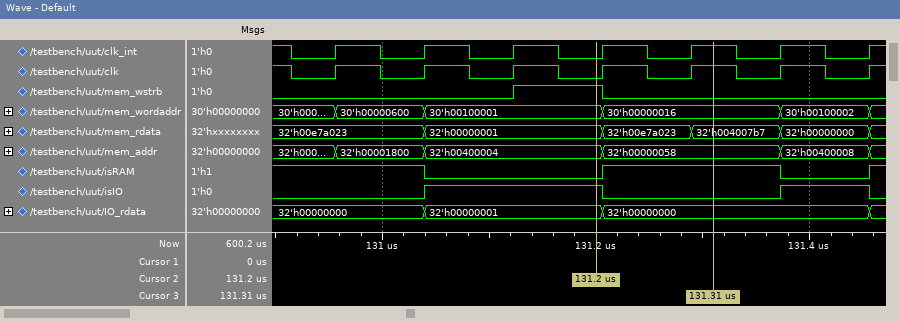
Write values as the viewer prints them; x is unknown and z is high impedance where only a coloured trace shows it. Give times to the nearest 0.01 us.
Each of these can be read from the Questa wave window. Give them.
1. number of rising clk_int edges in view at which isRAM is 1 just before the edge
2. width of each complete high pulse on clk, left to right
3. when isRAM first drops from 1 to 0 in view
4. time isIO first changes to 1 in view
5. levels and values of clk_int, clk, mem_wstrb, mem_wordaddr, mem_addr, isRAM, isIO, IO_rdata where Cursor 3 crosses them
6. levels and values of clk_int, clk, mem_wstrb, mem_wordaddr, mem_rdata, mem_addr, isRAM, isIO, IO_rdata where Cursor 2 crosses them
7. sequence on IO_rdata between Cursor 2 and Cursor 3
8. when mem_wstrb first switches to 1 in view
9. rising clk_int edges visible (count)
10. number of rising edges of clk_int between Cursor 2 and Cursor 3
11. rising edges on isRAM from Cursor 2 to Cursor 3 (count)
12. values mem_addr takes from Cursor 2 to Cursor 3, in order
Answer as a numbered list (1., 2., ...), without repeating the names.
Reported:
1. 4
2. 0.04 us, 0.04 us, 0.04 us, 0.04 us, 0.04 us, 0.04 us
3. 131.04 us
4. 131.04 us
5. clk_int=1, clk=1, mem_wstrb=0, mem_wordaddr=30'h00000016, mem_addr=32'h00000058, isRAM=1, isIO=0, IO_rdata=32'h00000000
6. clk_int=0, clk=0, mem_wstrb=1, mem_wordaddr=30'h00100001, mem_rdata=32'h00000001, mem_addr=32'h00400004, isRAM=0, isIO=1, IO_rdata=32'h00000001
7. 32'h00000001, 32'h00000000
8. 131.12 us
9. 7
10. 2
11. 1
12. 32'h00400004, 32'h00000058
